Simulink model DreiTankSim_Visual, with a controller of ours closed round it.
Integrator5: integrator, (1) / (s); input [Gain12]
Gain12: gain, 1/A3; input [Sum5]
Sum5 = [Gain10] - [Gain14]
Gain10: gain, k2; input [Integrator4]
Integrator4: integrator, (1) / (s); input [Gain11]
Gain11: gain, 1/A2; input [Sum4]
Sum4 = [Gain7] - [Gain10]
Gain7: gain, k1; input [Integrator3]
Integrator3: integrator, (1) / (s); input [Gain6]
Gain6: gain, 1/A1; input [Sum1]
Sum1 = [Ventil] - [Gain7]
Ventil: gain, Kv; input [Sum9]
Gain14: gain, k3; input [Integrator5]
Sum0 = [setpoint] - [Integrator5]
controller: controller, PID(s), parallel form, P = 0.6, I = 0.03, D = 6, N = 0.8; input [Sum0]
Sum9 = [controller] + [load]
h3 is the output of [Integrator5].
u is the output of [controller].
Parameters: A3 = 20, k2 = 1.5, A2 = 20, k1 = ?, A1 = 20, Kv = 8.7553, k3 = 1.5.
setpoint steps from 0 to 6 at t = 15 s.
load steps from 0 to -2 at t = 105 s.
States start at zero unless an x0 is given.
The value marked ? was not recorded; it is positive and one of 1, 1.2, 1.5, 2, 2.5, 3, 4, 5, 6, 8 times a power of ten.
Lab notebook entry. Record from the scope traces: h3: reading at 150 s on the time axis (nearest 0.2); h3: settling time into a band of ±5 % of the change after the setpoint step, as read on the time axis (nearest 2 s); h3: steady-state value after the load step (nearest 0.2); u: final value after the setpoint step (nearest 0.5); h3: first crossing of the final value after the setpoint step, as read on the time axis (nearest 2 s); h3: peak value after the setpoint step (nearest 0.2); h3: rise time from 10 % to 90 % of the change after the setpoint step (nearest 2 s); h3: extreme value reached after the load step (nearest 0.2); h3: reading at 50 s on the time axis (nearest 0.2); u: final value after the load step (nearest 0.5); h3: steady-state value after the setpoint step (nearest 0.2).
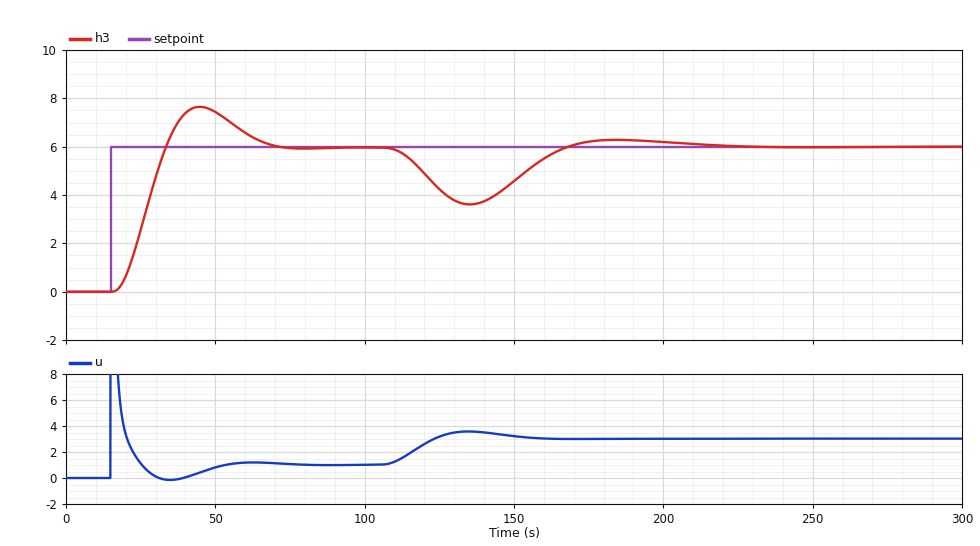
4.6
64 s
6.0
1.0
34 s
7.6
12 s
3.6
7.4
3.0
6.0
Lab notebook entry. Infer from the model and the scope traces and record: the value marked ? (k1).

1.5
